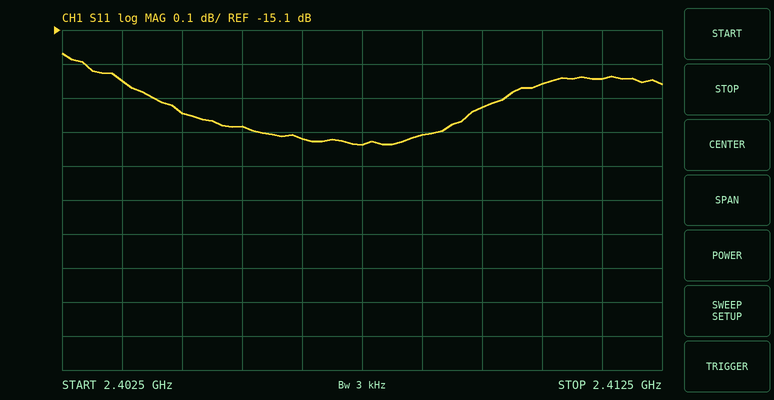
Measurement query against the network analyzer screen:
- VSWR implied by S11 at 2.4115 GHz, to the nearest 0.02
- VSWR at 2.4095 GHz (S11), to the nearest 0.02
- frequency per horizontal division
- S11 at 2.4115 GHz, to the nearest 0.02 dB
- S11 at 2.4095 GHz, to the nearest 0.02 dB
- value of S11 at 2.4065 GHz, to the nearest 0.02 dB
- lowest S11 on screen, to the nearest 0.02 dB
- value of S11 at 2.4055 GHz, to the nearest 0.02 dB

1.42
1.42
1 MHz
-15.24 dB
-15.32 dB
-15.42 dB
-15.44 dB
-15.38 dB
